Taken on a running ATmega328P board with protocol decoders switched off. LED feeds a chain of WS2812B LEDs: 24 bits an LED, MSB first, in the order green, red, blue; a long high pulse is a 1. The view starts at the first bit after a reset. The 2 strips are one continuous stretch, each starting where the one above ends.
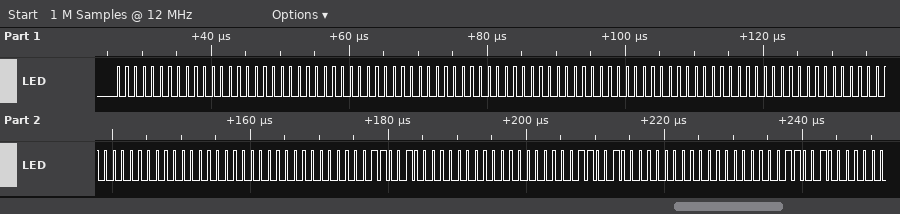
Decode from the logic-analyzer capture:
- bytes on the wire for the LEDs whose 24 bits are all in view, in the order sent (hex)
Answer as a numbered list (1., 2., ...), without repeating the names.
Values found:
1. 00 00 00 00 00 00 00 00 00 00 00 00 00 00 00 64 00 00 64 00 00
